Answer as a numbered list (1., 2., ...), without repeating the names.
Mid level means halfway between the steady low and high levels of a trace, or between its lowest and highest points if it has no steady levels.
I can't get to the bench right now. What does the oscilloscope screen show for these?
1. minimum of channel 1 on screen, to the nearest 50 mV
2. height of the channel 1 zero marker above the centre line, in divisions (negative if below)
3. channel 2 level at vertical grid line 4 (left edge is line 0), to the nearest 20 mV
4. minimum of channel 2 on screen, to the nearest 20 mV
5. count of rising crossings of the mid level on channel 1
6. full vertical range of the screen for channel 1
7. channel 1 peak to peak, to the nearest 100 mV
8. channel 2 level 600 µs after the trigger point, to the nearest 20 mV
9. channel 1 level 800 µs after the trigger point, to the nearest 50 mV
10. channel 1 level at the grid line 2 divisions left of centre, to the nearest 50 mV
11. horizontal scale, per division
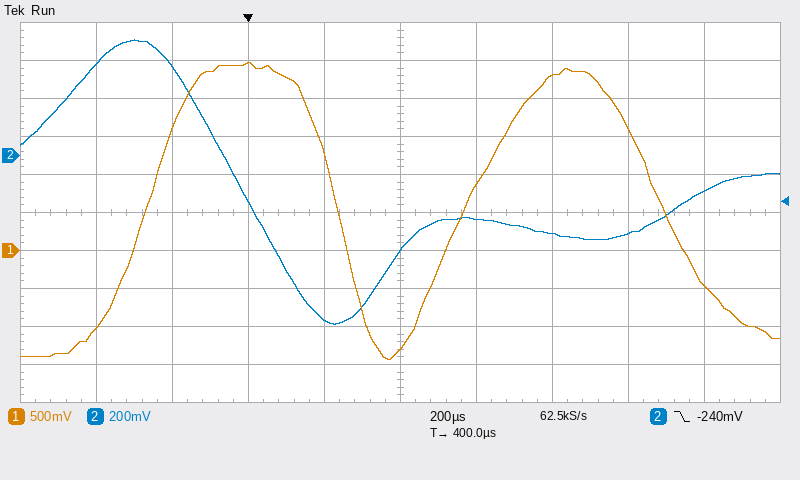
1. -1.45 V
2. -1.0 div
3. -860 mV
4. -880 mV
5. 2
6. 5 V
7. 3.90 V
8. -340 mV
9. 2.30 V
10. 2.45 V
11. 200 µs
